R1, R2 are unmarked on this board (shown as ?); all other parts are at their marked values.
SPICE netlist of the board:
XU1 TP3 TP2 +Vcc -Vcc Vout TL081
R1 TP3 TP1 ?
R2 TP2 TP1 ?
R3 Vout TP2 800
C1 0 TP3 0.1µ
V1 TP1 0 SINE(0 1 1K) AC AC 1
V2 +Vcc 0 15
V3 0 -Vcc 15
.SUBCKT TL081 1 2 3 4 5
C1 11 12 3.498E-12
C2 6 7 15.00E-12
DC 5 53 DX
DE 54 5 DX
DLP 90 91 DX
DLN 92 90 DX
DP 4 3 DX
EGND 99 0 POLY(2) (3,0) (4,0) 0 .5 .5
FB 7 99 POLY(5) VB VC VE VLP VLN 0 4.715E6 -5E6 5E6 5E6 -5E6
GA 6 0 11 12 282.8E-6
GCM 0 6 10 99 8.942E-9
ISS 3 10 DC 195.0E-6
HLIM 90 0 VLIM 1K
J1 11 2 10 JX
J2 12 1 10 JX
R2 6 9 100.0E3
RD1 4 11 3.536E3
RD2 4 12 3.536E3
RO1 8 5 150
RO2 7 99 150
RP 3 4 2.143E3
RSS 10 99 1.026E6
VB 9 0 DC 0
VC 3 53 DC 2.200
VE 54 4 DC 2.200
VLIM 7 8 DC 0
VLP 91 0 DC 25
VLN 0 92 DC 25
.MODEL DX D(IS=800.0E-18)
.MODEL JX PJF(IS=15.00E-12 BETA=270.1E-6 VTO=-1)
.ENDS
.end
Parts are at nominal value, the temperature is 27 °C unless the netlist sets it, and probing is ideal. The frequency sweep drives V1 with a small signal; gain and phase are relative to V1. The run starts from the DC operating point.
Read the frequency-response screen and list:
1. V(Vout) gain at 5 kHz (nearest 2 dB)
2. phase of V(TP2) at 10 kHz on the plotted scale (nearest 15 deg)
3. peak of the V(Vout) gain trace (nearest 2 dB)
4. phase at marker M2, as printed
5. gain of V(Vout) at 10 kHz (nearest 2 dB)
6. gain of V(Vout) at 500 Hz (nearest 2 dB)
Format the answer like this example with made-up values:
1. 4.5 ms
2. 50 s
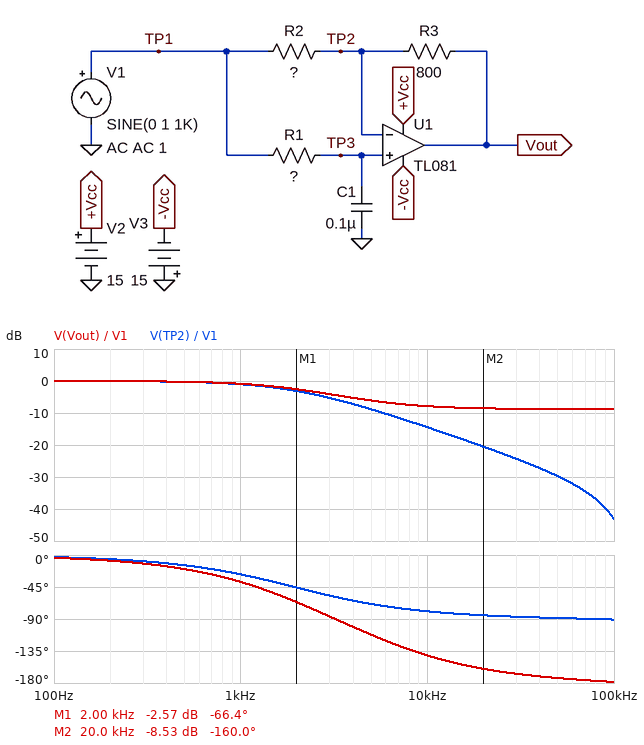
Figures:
1. -6 dB
2. -75 deg
3. 0 dB
4. -160.0 deg
5. -8 dB
6. 0 dB
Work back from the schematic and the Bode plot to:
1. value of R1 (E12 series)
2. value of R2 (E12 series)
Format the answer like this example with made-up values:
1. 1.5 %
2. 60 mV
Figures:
1. 820 Ω
2. 2.2 kΩ
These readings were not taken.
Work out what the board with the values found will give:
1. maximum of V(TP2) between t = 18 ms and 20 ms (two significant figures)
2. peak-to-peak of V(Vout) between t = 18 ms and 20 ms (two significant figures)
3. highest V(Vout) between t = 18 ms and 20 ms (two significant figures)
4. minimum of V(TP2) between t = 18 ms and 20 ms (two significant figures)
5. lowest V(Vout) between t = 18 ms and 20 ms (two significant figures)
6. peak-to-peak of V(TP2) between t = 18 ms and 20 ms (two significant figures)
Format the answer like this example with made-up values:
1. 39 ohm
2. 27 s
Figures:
1. 890 mV
2. 1.8 V
3. 900 mV
4. -890 mV
5. -900 mV
6. 1.8 V
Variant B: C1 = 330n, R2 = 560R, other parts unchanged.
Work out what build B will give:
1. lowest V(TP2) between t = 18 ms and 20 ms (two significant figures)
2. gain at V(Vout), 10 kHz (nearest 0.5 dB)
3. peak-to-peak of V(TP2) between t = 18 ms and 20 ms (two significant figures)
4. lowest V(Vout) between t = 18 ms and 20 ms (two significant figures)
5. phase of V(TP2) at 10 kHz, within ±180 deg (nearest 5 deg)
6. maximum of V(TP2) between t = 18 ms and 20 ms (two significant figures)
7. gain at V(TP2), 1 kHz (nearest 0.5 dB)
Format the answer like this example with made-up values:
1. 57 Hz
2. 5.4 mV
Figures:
1. -510 mV
2. 3.0 dB
3. 1.0 V
4. -1.3 V
5. -85 deg
6. 510 mV
7. -6.0 dB
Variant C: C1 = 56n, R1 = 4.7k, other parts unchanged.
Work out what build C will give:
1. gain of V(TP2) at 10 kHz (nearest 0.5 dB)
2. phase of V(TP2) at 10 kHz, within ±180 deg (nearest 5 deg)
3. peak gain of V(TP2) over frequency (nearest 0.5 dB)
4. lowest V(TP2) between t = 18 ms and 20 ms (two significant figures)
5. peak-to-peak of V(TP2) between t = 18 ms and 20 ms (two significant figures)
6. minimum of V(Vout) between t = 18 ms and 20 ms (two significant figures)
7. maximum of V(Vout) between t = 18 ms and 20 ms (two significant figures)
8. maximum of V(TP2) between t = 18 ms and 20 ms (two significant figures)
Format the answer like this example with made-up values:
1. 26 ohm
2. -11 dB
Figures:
1. -24.5 dB
2. -85 deg
3. 0 dB
4. -520 mV
5. 1.0 V
6. -600 mV
7. 600 mV
8. 520 mV
